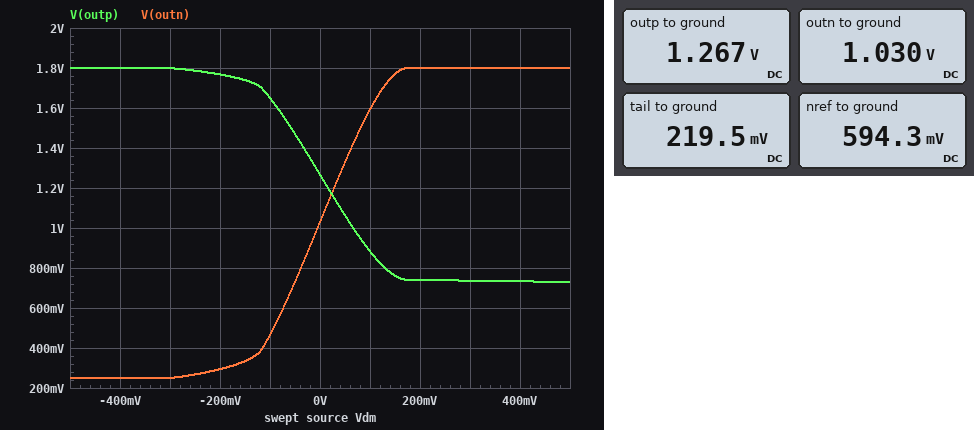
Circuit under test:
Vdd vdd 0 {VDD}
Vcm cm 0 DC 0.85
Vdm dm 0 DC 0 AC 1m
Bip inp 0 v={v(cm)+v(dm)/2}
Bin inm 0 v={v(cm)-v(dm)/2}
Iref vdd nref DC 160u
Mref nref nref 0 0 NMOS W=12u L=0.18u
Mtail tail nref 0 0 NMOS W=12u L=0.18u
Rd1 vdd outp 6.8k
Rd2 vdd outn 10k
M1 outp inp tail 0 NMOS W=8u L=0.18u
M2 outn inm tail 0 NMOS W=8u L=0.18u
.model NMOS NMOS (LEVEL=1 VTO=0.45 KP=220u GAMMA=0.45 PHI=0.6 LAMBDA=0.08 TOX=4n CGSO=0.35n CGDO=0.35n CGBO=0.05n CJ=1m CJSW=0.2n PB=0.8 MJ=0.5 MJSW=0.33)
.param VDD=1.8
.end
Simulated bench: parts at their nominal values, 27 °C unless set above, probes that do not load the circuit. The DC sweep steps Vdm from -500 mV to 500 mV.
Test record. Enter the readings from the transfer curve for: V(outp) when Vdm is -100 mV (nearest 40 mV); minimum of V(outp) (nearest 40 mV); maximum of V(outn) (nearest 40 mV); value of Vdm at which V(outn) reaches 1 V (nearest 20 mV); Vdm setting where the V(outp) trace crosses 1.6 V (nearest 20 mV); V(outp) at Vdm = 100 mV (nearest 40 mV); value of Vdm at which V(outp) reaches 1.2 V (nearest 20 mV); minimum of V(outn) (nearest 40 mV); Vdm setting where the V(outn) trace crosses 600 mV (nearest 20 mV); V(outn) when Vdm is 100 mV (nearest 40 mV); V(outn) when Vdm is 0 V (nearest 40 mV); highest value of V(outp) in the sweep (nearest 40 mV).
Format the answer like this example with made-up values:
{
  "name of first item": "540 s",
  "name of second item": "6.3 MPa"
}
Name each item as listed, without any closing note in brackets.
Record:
{
  "V(outp) when Vdm is -100 mV": "1.64 V",
  "minimum of V(outp)": "720 mV",
  "maximum of V(outn)": "1.80 V",
  "value of Vdm at which V(outn) reaches 1 V": "0 V",
  "Vdm setting where the V(outp) trace crosses 1.6 V": "-80 mV",
  "V(outp) at Vdm = 100 mV": "880 mV",
  "value of Vdm at which V(outp) reaches 1.2 V": "20 mV",
  "minimum of V(outn)": "240 mV",
  "Vdm setting where the V(outn) trace crosses 600 mV": "-80 mV",
  "V(outn) when Vdm is 100 mV": "1.60 V",
  "V(outn) when Vdm is 0 V": "1.04 V",
  "highest value of V(outp) in the sweep": "1.80 V"
}
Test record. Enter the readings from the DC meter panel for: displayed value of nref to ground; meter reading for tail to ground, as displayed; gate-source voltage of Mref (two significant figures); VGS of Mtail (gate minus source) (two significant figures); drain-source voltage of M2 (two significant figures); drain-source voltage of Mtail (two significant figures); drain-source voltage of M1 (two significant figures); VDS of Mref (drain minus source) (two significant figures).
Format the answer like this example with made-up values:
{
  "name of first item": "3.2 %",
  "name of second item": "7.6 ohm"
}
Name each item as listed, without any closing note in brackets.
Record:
{
  "displayed value of nref to ground": "594.3 mV",
  "meter reading for tail to ground, as displayed": "219.5 mV",
  "gate-source voltage of Mref": "590 mV",
  "VGS of Mtail (gate minus source)": "590 mV",
  "drain-source voltage of M2": "810 mV",
  "drain-source voltage of Mtail": "220 mV",
  "drain-source voltage of M1": "1.0 V",
  "VDS of Mref (drain minus source)": "590 mV"
}
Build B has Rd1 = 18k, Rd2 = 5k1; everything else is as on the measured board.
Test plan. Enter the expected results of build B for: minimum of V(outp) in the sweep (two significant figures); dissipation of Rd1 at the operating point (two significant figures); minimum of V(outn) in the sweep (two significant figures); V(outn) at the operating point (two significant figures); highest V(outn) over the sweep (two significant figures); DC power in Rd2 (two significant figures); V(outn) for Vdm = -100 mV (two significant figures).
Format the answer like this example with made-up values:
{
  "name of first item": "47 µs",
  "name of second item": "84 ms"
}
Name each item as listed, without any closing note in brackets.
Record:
{
  "minimum of V(outp) in the sweep": "89 mV",
  "dissipation of Rd1 at the operating point": "100 µW",
  "minimum of V(outn) in the sweep": "1.0 V",
  "V(outn) at the operating point": "1.4 V",
  "highest V(outn) over the sweep": "1.7 V",
  "DC power in Rd2": "33 µW",
  "V(outn) for Vdm = -100 mV": "1.1 V"
}
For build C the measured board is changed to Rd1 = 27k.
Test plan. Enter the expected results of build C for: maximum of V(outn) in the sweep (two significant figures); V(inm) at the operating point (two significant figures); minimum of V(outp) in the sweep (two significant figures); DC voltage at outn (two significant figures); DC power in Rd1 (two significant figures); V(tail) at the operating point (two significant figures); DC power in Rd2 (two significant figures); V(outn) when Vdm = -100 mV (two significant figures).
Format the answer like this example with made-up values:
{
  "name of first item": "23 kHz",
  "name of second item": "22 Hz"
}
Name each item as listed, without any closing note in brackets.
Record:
{
  "maximum of V(outn) in the sweep": "1.5 V",
  "V(inm) at the operating point": "850 mV",
  "minimum of V(outp) in the sweep": "68 mV",
  "DC voltage at outn": "820 mV",
  "DC power in Rd1": "88 µW",
  "V(tail) at the operating point": "210 mV",
  "DC power in Rd2": "96 µW",
  "V(outn) when Vdm = -100 mV": "460 mV"
}
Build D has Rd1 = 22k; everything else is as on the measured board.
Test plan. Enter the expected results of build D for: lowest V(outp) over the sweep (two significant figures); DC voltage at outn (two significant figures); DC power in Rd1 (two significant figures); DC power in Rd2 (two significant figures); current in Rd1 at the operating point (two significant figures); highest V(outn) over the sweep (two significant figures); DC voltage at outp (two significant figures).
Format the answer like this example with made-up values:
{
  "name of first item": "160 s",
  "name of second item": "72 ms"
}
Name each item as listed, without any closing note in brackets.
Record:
{
  "lowest V(outp) over the sweep": "77 mV",
  "DC voltage at outn": "930 mV",
  "DC power in Rd1": "100 µW",
  "DC power in Rd2": "75 µW",
  "current in Rd1 at the operating point": "69 µA",
  "highest V(outn) over the sweep": "1.5 V",
  "DC voltage at outp": "290 mV"
}
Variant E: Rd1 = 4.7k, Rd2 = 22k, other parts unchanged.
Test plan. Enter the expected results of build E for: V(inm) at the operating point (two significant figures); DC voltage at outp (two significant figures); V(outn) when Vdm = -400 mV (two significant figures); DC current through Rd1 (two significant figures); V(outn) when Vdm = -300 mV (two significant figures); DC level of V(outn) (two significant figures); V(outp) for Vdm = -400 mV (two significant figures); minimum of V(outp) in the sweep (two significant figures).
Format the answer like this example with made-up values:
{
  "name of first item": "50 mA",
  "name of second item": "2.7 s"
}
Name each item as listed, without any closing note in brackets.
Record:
{
  "V(inm) at the operating point": "850 mV",
  "DC voltage at outp": "1.4 V",
  "V(outn) when Vdm = -400 mV": "99 mV",
  "DC current through Rd1": "87 µA",
  "V(outn) when Vdm = -300 mV": "130 mV",
  "DC level of V(outn)": "290 mV",
  "V(outp) for Vdm = -400 mV": "1.6 V",
  "minimum of V(outp) in the sweep": "1.1 V"
}
